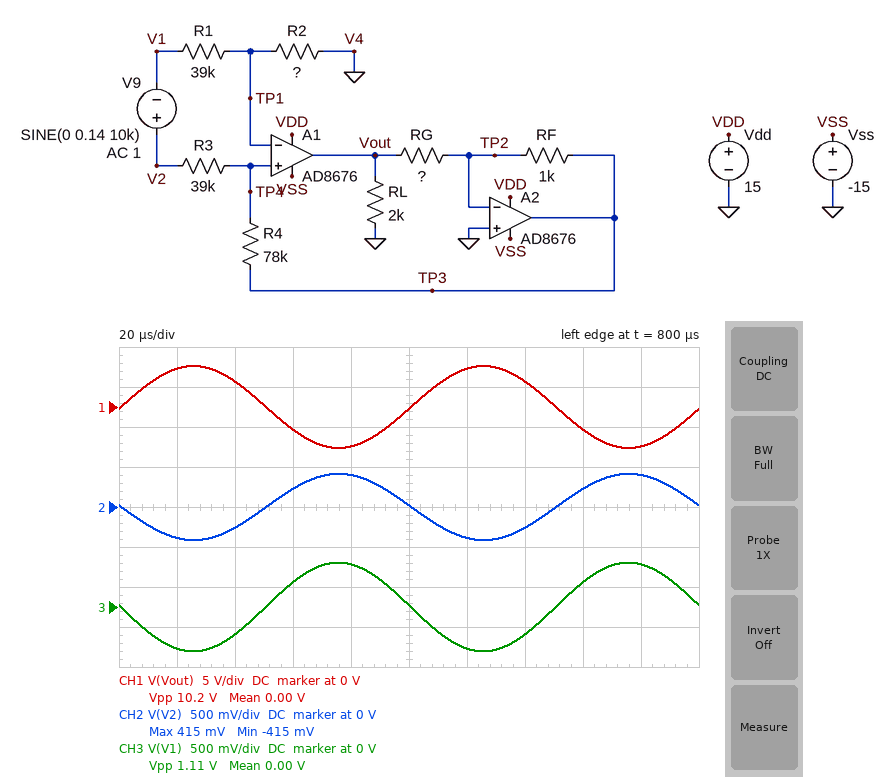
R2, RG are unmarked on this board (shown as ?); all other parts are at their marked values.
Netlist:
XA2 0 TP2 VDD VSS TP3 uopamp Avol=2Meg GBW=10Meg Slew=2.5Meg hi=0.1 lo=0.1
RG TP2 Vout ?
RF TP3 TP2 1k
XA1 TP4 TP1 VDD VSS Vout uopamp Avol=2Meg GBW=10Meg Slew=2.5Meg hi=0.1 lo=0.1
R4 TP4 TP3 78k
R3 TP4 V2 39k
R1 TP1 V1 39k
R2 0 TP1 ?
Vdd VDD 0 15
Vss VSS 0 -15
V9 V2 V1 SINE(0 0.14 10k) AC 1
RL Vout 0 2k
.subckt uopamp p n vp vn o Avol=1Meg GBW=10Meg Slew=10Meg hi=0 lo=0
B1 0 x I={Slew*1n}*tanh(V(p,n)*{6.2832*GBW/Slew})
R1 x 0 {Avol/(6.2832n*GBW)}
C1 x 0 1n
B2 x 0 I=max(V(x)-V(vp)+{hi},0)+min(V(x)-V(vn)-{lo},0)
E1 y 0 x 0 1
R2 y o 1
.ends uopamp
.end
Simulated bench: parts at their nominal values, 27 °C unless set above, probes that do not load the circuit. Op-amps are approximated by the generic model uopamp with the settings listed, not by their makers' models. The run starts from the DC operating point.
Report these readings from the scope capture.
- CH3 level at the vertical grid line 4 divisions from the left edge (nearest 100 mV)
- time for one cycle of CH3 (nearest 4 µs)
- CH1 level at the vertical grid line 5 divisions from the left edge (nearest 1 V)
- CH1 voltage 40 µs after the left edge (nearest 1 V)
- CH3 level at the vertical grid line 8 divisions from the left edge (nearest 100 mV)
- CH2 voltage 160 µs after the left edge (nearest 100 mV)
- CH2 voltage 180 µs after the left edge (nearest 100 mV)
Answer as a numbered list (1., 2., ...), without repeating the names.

1. 500 mV
2. 100 µs
3. 0 V
4. 3 V
5. 300 mV
6. 200 mV
7. 400 mV
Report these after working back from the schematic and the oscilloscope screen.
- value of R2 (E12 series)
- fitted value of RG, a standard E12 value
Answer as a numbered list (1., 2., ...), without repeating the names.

1. 270 kΩ
2. 8.2 kΩ
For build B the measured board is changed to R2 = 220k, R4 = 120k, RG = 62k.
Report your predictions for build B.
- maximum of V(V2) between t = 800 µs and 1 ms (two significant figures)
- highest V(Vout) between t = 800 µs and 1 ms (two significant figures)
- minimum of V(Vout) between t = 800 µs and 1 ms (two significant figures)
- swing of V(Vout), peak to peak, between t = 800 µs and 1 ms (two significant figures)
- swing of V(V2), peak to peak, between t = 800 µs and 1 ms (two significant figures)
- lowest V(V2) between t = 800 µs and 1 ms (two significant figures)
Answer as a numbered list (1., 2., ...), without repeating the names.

1. 130 mV
2. 15 V
3. -15 V
4. 30 V
5. 260 mV
6. -130 mV
